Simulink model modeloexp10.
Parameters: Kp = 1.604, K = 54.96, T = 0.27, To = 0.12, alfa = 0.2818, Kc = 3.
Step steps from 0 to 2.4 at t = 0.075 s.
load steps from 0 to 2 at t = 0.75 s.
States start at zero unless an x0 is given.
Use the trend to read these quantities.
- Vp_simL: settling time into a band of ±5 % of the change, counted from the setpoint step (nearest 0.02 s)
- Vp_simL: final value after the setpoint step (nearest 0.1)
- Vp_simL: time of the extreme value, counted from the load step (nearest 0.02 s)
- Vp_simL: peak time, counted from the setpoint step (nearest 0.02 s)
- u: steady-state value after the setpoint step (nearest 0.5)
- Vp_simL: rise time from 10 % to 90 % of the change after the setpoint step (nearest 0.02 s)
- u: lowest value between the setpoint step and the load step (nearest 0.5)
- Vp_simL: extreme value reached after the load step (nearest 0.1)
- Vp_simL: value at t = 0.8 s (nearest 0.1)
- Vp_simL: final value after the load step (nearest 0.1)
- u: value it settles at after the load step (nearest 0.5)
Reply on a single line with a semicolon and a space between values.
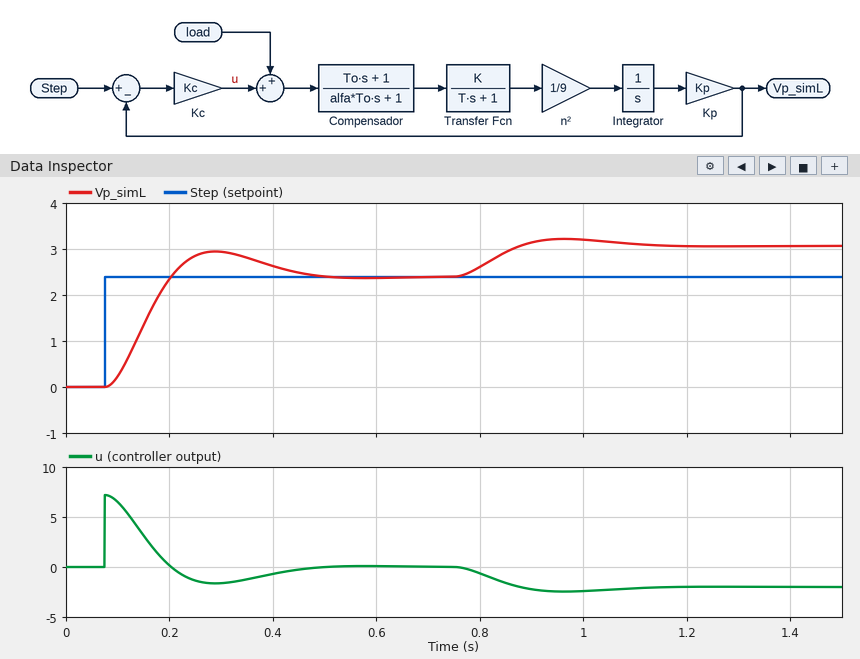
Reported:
0.36 s; 2.4; 0.22 s; 0.22 s; 0.0; 0.08 s; -1.5; 3.2; 2.6; 3.1; -2.0
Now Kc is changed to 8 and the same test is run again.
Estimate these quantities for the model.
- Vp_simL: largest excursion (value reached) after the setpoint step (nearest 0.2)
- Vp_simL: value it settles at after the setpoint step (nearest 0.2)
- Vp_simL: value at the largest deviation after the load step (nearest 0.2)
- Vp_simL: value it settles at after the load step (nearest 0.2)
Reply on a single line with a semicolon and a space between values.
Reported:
3.2; 2.4; 2.8; 2.6
